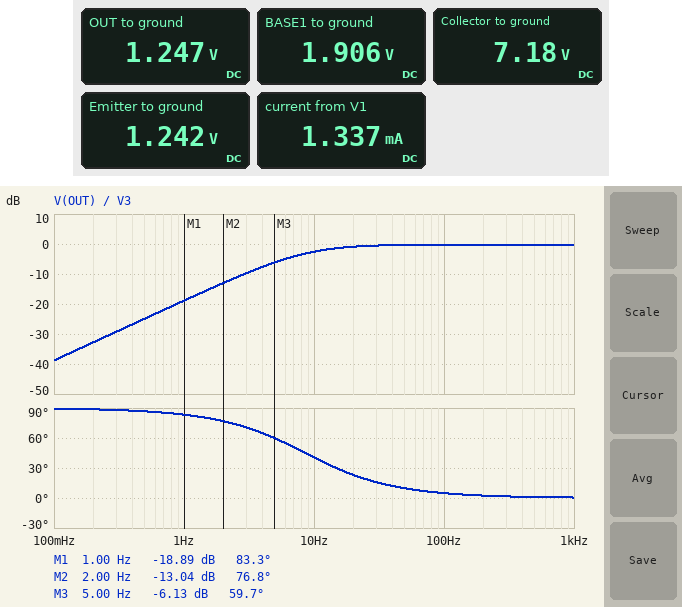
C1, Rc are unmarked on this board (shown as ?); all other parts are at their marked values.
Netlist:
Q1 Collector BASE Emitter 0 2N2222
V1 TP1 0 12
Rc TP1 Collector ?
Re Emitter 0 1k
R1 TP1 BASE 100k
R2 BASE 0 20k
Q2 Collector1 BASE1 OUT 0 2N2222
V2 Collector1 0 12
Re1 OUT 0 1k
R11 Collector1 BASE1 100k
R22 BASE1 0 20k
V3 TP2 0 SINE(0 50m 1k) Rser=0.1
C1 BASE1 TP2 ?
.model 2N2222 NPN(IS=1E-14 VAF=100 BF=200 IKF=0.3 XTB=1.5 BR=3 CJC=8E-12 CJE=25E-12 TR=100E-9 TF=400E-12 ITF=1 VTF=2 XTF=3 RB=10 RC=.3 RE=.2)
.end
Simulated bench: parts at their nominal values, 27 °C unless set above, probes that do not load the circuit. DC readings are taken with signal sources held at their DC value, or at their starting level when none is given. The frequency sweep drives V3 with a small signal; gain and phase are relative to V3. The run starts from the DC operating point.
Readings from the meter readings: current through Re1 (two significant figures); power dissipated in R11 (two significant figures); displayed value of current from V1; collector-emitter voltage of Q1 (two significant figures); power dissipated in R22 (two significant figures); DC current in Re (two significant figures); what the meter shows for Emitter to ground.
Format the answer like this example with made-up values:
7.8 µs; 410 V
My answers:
1.2 mA; 1.0 mW; 1.337 mA; 5.9 V; 180 µW; 1.2 mA; 1.242 V
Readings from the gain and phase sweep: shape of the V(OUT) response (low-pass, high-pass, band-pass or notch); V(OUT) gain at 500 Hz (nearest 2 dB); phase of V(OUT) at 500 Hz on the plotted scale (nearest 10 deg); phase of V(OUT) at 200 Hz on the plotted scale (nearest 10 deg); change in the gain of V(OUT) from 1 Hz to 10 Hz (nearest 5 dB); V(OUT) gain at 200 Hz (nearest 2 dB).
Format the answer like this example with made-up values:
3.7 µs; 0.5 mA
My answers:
high-pass; 0 dB; 0 deg; 0 deg; 15 dB; 0 dB
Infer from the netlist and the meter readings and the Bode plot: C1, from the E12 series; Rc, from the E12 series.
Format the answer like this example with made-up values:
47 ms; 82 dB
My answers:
1.2 µF; 3.9 kΩ
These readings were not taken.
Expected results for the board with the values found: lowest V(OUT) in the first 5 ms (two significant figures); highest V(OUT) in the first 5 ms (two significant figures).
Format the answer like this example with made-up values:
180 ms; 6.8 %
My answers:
1.2 V; 1.3 V
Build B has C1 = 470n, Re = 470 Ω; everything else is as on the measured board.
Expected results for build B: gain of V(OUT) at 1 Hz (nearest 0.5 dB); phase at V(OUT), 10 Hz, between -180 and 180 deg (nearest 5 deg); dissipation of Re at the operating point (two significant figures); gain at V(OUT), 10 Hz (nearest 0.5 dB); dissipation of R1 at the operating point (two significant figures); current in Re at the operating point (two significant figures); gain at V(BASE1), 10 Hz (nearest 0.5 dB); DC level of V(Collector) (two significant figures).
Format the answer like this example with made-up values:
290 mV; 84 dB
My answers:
-27.0 dB; 65 deg; 2.7 mW; -8.0 dB; 1.0 mW; 2.4 mA; -7.5 dB; 2.7 V
